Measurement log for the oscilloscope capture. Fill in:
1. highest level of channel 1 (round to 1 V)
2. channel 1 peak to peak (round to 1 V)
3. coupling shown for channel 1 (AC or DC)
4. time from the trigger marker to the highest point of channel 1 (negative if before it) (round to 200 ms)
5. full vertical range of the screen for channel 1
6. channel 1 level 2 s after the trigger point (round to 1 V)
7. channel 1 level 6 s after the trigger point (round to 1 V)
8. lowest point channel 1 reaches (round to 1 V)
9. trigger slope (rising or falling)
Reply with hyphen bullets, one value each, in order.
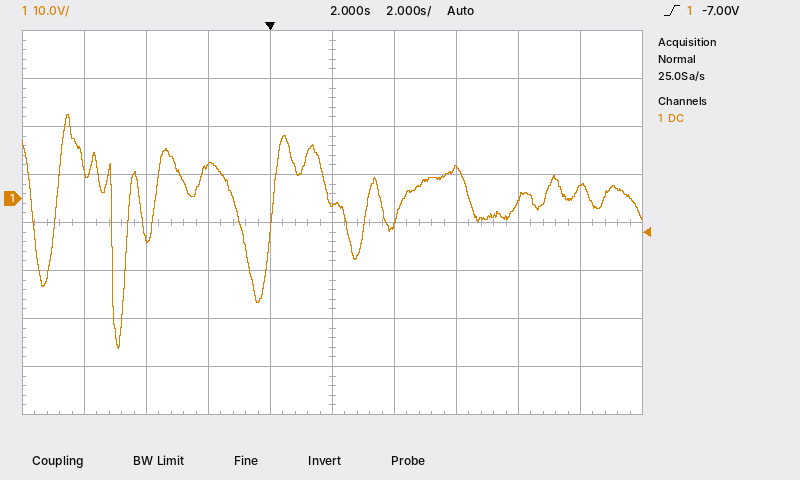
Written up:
- 18 V
- 49 V
- DC
- -6.6 s
- 80 V
- -1 V
- 6 V
- -31 V
- rising
